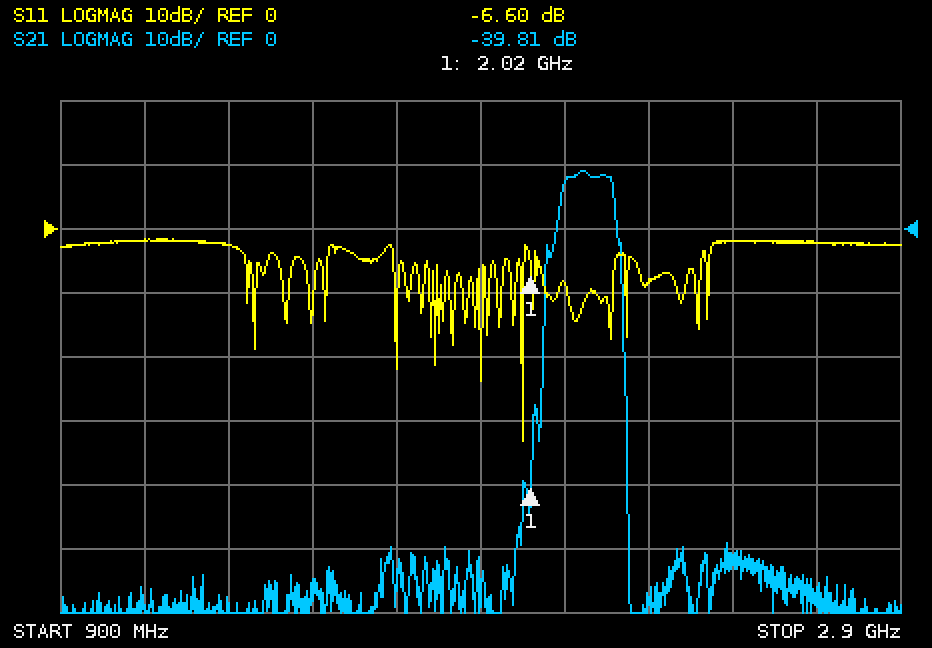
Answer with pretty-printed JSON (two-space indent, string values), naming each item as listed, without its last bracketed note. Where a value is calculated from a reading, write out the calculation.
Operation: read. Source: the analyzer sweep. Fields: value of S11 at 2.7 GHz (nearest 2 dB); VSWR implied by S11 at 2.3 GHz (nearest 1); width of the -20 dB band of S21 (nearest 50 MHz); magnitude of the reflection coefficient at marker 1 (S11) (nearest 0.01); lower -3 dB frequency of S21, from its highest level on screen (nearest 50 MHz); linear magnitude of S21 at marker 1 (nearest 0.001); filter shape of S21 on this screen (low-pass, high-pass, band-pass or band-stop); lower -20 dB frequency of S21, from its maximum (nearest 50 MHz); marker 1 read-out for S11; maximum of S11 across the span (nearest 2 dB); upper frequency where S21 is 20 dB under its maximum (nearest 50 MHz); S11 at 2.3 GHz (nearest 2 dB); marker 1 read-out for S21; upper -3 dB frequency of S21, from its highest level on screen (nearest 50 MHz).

{
  "value of S11 at 2.7 GHz": "-2 dB",
  "VSWR implied by S11 at 2.3 GHz": "|Γ| = 10^(-8/20) = 0.3981; VSWR = (1 + 0.3981)/(1 − 0.3981) ≈ 2",
  "width of the -20 dB band of S21": "2.25 GHz − 2.05 GHz = 200 MHz",
  "magnitude of the reflection coefficient at marker 1 (S11)": "10^(-6.6/20) ≈ 0.47",
  "lower -3 dB frequency of S21, from its highest level on screen": "2.10 GHz",
  "linear magnitude of S21 at marker 1": "10^(-39.81/20) ≈ 0.010",
  "filter shape of S21 on this screen": "band-pass",
  "lower -20 dB frequency of S21, from its maximum": "2.05 GHz",
  "marker 1 read-out for S11": "-6.60 dB",
  "maximum of S11 across the span": "-2 dB",
  "upper frequency where S21 is 20 dB under its maximum": "2.25 GHz",
  "S11 at 2.3 GHz": "-8 dB",
  "marker 1 read-out for S21": "-39.81 dB",
  "upper -3 dB frequency of S21, from its highest level on screen": "2.20 GHz"
}
